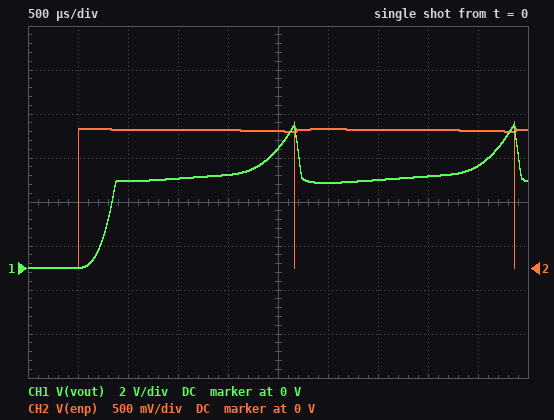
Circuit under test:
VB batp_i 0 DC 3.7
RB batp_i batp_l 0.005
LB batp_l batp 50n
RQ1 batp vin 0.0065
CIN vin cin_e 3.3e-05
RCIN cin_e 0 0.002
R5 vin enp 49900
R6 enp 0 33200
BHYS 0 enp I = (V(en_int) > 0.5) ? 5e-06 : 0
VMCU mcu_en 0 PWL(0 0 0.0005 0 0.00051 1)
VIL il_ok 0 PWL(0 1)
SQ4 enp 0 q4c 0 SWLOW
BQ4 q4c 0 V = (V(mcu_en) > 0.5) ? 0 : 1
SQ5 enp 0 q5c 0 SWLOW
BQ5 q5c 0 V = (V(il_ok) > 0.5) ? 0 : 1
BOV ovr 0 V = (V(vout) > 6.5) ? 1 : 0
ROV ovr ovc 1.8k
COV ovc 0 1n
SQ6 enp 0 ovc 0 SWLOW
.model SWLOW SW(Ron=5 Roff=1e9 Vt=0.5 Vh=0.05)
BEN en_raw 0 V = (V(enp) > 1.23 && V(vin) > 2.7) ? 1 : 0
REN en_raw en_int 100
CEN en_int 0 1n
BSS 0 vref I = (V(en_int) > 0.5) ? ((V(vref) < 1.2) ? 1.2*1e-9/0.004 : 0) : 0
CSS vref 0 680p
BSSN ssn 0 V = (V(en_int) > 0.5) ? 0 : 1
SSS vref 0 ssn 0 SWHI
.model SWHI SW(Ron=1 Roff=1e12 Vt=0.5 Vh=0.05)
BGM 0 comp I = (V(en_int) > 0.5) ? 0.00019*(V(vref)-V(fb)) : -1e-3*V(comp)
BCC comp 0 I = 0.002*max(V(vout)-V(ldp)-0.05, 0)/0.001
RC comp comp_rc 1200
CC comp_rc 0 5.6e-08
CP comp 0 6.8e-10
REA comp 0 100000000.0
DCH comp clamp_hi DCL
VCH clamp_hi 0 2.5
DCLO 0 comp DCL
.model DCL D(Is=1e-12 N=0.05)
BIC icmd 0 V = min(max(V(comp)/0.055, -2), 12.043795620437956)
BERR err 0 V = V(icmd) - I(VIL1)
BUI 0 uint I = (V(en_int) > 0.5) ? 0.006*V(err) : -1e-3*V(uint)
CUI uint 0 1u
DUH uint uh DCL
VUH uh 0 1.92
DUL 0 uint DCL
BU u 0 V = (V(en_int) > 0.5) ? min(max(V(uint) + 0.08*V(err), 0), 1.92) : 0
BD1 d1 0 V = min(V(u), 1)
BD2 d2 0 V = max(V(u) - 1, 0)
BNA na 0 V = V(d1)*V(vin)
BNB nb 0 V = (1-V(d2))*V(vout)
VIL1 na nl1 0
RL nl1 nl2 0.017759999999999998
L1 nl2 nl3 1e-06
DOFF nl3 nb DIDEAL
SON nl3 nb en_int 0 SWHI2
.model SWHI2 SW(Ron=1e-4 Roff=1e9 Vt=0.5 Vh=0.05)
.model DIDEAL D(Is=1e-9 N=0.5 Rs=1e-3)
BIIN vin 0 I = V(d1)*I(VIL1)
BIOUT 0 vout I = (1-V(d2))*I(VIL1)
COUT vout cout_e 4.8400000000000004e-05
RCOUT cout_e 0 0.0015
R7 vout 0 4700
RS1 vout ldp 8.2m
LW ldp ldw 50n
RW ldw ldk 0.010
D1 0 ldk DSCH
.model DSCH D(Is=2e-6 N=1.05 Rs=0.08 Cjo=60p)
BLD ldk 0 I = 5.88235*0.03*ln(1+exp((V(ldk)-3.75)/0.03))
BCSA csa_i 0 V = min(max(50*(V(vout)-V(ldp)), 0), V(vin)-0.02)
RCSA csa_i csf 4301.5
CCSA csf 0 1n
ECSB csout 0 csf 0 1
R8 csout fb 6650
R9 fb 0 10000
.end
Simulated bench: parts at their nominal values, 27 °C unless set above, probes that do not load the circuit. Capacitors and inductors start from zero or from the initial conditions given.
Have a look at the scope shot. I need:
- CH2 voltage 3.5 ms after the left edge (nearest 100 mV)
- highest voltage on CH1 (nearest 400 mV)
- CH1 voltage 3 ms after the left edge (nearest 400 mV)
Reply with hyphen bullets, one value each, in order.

- 1.6 V
- 6.4 V
- 4.0 V
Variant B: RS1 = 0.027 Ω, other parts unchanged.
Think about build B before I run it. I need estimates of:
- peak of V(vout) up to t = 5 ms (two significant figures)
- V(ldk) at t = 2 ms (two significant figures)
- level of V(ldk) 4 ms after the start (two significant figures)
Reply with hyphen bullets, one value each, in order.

- 4.1 V
- 3.9 V
- 4.0 V
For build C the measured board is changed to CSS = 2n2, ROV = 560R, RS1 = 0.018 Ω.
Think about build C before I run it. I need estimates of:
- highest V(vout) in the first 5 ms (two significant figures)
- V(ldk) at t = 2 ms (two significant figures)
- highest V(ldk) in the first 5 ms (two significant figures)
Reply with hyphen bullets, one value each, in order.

- 4.0 V
- 3.8 V
- 3.9 V
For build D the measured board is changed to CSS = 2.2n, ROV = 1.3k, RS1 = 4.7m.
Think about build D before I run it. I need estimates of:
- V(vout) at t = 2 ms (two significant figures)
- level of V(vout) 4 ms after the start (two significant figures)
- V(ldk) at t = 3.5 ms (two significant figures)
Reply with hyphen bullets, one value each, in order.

- 4.0 V
- 5.0 V
- 4.3 V
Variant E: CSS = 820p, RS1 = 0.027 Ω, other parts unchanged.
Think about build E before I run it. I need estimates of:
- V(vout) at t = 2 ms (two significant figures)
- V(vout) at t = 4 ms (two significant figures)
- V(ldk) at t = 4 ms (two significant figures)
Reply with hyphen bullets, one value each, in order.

- 3.9 V
- 4.1 V
- 4.0 V
